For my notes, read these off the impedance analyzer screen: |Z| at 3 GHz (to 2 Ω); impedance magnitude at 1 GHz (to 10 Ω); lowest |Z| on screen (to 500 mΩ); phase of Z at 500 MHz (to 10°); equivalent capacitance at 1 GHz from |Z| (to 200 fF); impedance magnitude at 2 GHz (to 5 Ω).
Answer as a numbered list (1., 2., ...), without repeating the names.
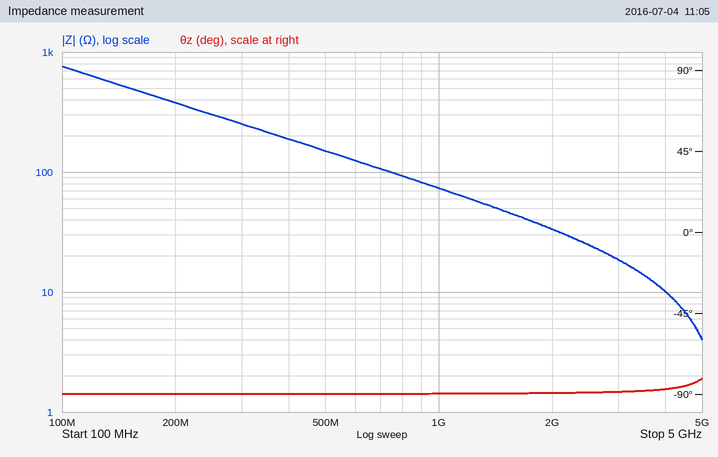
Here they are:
1. 18 Ω
2. 70 Ω
3. 4.0 Ω
4. -90°
5. 2.2 pF
6. 35 Ω
